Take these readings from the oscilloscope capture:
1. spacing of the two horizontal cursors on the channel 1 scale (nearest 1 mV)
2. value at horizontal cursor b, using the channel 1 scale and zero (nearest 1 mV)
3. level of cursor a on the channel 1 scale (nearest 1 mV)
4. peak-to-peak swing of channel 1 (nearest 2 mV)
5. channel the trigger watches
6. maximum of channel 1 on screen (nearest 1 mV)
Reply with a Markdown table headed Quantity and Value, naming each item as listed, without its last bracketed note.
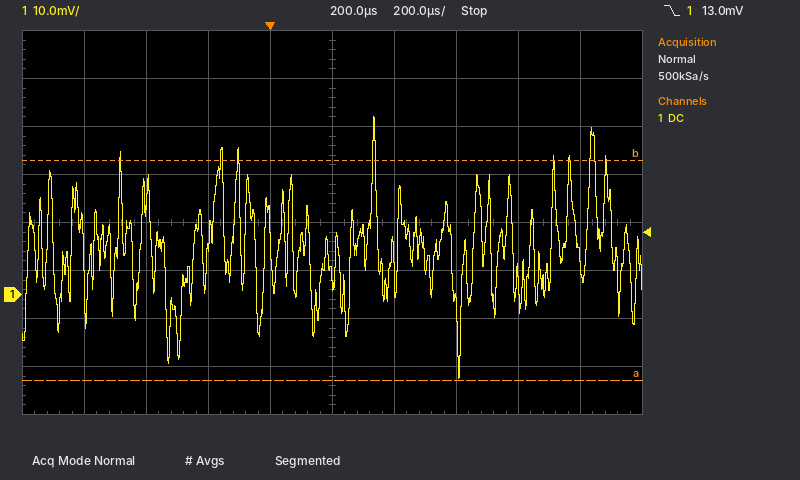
| Quantity | Value |
|---|---|
| spacing of the two horizontal cursors on the channel 1 scale | 46 mV |
| value at horizontal cursor b, using the channel 1 scale and zero | 28 mV |
| level of cursor a on the channel 1 scale | -18 mV |
| peak-to-peak swing of channel 1 | 54 mV |
| channel the trigger watches | channel 1 |
| maximum of channel 1 on screen | 37 mV |
